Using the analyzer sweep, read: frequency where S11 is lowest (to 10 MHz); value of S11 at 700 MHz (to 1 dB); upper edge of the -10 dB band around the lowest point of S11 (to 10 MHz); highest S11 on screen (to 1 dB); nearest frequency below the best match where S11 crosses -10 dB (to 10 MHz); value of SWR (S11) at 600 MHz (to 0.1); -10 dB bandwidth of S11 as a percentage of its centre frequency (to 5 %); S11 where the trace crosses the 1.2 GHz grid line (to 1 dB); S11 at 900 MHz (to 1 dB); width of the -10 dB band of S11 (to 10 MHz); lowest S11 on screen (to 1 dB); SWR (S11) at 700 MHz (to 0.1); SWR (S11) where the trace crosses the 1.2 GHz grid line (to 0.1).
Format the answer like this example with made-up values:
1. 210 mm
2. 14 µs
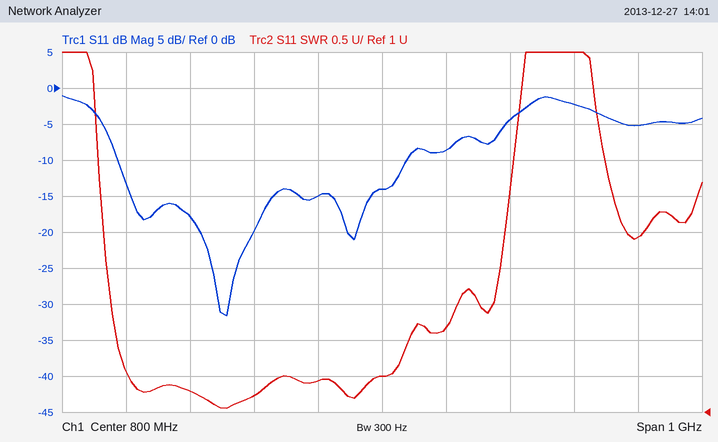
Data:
1. 560 MHz
2. -15 dB
3. 840 MHz
4. -1 dB
5. 390 MHz
6. 1.2
7. 75 %
8. -5 dB
9. -9 dB
10. 450 MHz
11. -32 dB
12. 1.4
13. 3.4
